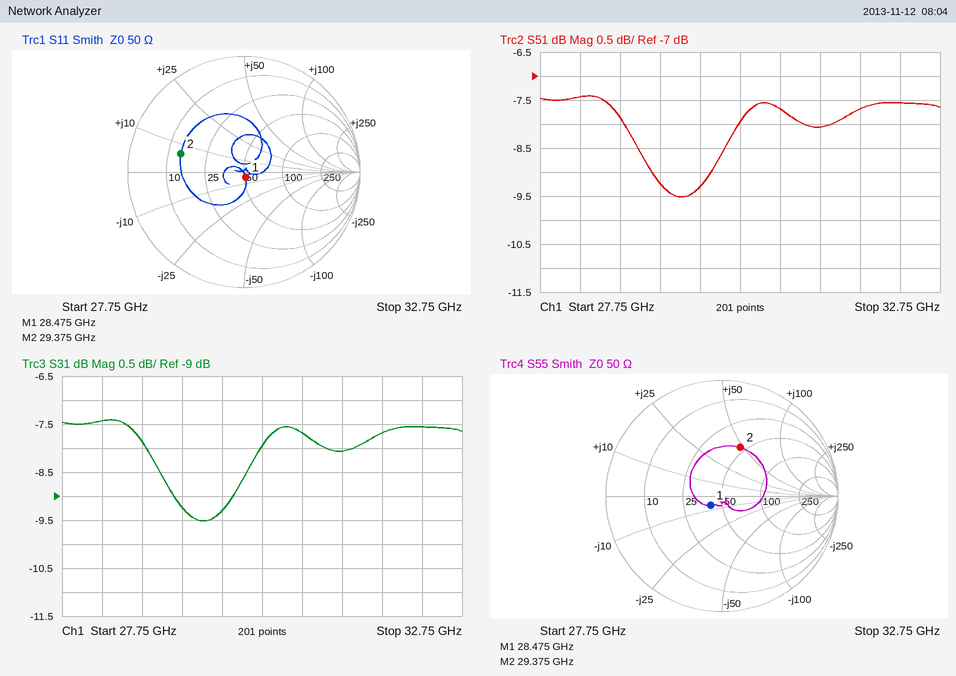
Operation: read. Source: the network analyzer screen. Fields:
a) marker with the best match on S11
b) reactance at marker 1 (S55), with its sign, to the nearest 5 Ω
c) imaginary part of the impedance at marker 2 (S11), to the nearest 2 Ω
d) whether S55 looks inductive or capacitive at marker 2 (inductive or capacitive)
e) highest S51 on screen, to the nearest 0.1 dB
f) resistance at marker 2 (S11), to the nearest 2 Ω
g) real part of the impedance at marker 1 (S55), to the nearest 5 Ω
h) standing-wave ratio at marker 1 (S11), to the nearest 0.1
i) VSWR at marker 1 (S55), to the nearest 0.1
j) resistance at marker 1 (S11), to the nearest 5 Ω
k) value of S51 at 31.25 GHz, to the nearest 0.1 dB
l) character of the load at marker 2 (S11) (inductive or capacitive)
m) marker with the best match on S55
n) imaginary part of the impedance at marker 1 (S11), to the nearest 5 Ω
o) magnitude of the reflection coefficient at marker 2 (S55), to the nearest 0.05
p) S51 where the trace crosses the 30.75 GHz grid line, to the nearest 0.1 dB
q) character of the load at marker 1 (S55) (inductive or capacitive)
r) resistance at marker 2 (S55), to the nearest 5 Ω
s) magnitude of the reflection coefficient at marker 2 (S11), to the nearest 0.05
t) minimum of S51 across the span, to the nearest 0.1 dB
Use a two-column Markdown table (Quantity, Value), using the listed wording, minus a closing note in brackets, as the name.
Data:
| Quantity | Value |
|---|---|
| marker with the best match on S11 | marker 1 |
| reactance at marker 1 (S55), with its sign, to the nearest 5 Ω | -5 Ω |
| imaginary part of the impedance at marker 2 (S11), to the nearest 2 Ω | +6 Ω |
| whether S55 looks inductive or capacitive at marker 2 | inductive |
| highest S51 on screen, to the nearest 0.1 dB | -7.4 dB |
| resistance at marker 2 (S11), to the nearest 2 Ω | 14 Ω |
| real part of the impedance at marker 1 (S55), to the nearest 5 Ω | 40 Ω |
| standing-wave ratio at marker 1 (S11), to the nearest 0.1 | 1.1 |
| VSWR at marker 1 (S55), to the nearest 0.1 | 1.3 |
| resistance at marker 1 (S11), to the nearest 5 Ω | 50 Ω |
| value of S51 at 31.25 GHz, to the nearest 0.1 dB | -8.1 dB |
| character of the load at marker 2 (S11) | inductive |
| marker with the best match on S55 | marker 1 |
| imaginary part of the impedance at marker 1 (S11), to the nearest 5 Ω | -5 Ω |
| magnitude of the reflection coefficient at marker 2 (S55), to the nearest 0.05 | 0.45 |
| S51 where the trace crosses the 30.75 GHz grid line, to the nearest 0.1 dB | -7.7 dB |
| character of the load at marker 1 (S55) | capacitive |
| resistance at marker 2 (S55), to the nearest 5 Ω | 45 Ω |
| magnitude of the reflection coefficient at marker 2 (S11), to the nearest 0.05 | 0.55 |
| minimum of S51 across the span, to the nearest 0.1 dB | -9.5 dB |
